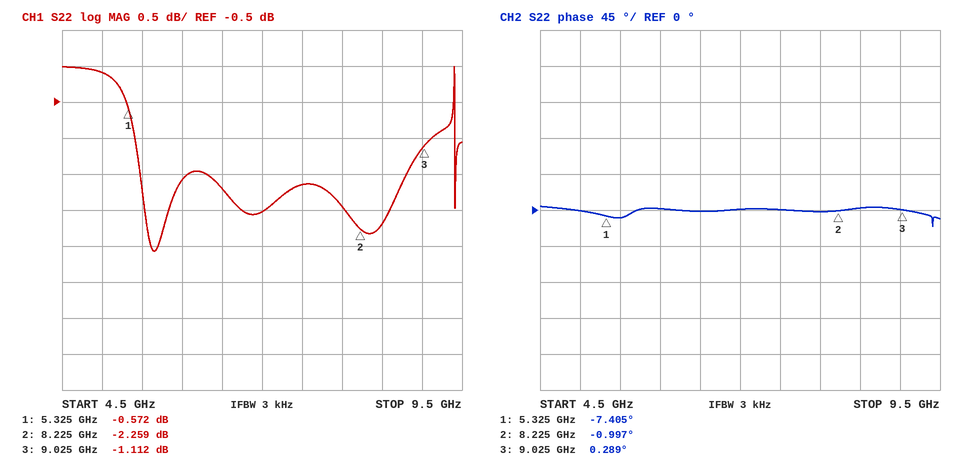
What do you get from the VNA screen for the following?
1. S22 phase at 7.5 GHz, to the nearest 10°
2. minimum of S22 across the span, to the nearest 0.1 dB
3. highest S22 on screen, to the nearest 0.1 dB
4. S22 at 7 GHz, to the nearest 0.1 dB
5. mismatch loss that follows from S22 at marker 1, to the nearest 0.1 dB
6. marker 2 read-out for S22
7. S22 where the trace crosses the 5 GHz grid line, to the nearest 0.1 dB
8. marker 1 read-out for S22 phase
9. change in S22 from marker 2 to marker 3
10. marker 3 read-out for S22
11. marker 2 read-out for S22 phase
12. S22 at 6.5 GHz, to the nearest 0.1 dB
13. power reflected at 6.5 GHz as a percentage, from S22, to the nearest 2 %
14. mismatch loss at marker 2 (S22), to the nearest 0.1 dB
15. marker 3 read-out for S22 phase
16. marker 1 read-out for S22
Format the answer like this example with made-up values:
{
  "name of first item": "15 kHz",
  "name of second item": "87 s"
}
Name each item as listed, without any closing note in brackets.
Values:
{
  "S22 phase at 7.5 GHz, to the nearest 10°": "0°",
  "minimum of S22 across the span, to the nearest 0.1 dB": "-2.6 dB",
  "highest S22 on screen, to the nearest 0.1 dB": "0.0 dB",
  "S22 at 7 GHz, to the nearest 0.1 dB": "-2.0 dB",
  "mismatch loss that follows from S22 at marker 1, to the nearest 0.1 dB": "9.1 dB",
  "marker 2 read-out for S22": "-2.259 dB",
  "S22 where the trace crosses the 5 GHz grid line, to the nearest 0.1 dB": "-0.1 dB",
  "marker 1 read-out for S22 phase": "-7.405°",
  "change in S22 from marker 2 to marker 3": "1.147 dB",
  "marker 3 read-out for S22": "-1.112 dB",
  "marker 2 read-out for S22 phase": "-0.997°",
  "S22 at 6.5 GHz, to the nearest 0.1 dB": "-1.7 dB",
  "power reflected at 6.5 GHz as a percentage, from S22, to the nearest 2 %": "68 %",
  "mismatch loss at marker 2 (S22), to the nearest 0.1 dB": "3.9 dB",
  "marker 3 read-out for S22 phase": "0.289°",
  "marker 1 read-out for S22": "-0.572 dB"
}
